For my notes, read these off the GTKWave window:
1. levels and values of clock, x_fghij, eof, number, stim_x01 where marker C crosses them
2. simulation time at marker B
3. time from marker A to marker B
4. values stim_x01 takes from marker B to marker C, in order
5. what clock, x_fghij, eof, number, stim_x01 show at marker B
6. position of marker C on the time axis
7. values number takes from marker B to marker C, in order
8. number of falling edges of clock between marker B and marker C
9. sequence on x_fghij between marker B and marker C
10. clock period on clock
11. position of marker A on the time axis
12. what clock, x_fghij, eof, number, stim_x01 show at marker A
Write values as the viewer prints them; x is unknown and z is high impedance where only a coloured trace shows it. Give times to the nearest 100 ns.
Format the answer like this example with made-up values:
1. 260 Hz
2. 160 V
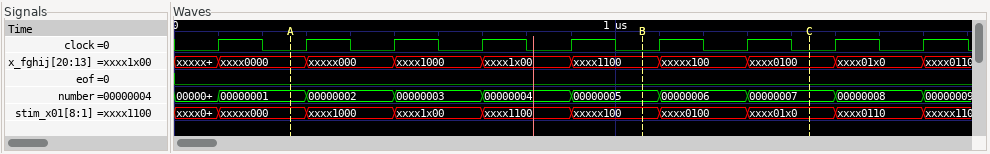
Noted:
1. clock=0, x_fghij=xxxx0100, eof=0, number=00000007, stim_x01=xxxx01x0
2. 1100 ns
3. 800 ns
4. xxxxx100, xxxx0100, xxxx01x0
5. clock=0, x_fghij=xxxx1100, eof=0, number=00000005, stim_x01=xxxxx100
6. 1400 ns
7. 00000005, 00000006, 00000007
8. 2
9. xxxx1100, xxxxx100, xxxx0100
10. 200 ns
11. 300 ns
12. clock=0, x_fghij=xxxx0000, eof=0, number=00000001, stim_x01=xxxxx000
